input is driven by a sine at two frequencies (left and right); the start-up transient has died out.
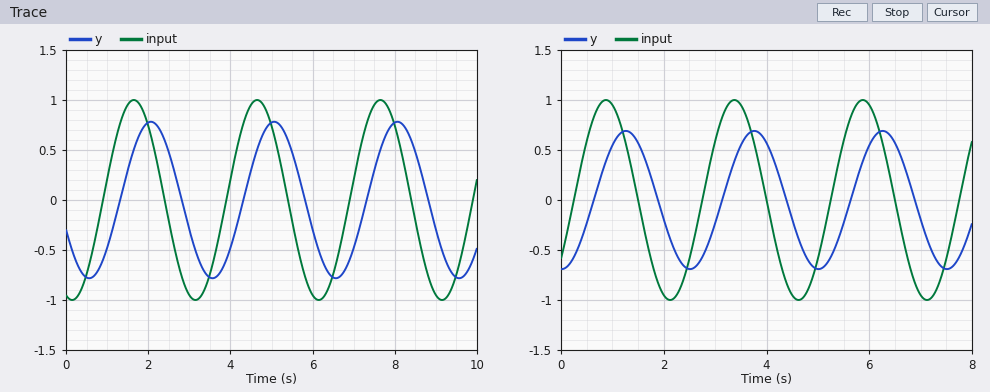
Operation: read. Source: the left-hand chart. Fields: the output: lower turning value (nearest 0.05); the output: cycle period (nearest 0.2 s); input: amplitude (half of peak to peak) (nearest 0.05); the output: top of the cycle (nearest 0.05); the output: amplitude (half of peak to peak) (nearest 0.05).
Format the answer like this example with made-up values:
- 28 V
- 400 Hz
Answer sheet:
- -0.80
- 3.0 s
- 1.00
- 0.80
- 0.80
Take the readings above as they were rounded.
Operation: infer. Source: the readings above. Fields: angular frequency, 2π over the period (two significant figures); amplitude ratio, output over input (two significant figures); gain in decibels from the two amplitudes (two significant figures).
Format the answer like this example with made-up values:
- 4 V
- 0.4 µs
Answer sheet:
- 2.1 rad/s
- 0.80
- -1.9 dB
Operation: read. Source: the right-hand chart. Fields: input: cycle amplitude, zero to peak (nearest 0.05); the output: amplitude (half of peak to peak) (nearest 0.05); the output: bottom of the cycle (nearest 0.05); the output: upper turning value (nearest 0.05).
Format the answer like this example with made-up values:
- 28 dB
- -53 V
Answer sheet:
- 1.00
- 0.70
- -0.70
- 0.70
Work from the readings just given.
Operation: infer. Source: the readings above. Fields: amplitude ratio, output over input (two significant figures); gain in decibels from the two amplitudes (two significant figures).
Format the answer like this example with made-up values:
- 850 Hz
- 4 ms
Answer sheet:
- 0.70
- -3.1 dB
